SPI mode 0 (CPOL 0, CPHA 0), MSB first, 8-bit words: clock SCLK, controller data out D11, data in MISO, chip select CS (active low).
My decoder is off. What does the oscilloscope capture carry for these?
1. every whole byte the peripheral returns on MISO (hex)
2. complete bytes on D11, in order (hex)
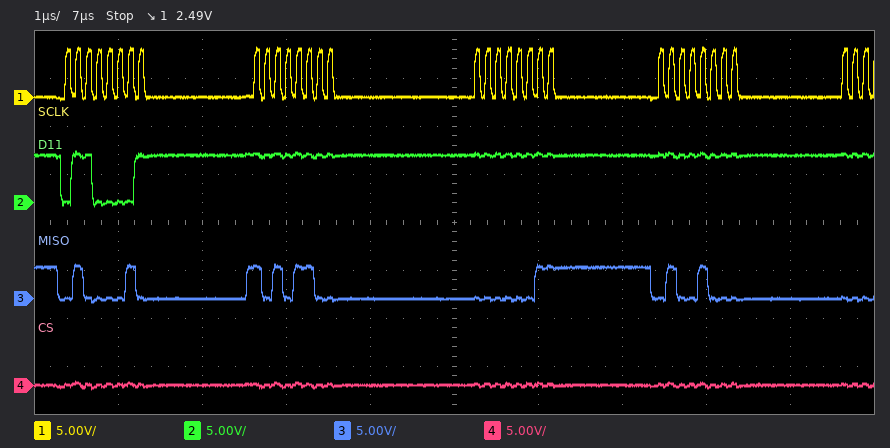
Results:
42 AC 03 48
61 FF FF FF
